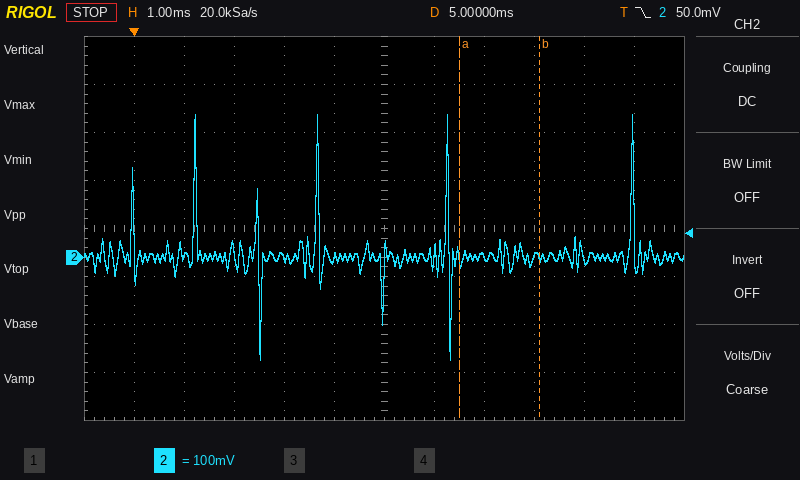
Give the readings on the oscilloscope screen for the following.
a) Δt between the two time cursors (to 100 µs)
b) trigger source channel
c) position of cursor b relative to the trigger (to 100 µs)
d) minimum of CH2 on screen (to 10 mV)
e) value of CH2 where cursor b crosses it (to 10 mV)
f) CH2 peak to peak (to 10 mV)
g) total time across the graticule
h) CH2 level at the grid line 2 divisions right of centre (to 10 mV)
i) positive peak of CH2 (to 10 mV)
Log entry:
1.6 ms
CH2
+8.1 ms
-210 mV
0 mV
510 mV
12 ms
0 mV
300 mV
